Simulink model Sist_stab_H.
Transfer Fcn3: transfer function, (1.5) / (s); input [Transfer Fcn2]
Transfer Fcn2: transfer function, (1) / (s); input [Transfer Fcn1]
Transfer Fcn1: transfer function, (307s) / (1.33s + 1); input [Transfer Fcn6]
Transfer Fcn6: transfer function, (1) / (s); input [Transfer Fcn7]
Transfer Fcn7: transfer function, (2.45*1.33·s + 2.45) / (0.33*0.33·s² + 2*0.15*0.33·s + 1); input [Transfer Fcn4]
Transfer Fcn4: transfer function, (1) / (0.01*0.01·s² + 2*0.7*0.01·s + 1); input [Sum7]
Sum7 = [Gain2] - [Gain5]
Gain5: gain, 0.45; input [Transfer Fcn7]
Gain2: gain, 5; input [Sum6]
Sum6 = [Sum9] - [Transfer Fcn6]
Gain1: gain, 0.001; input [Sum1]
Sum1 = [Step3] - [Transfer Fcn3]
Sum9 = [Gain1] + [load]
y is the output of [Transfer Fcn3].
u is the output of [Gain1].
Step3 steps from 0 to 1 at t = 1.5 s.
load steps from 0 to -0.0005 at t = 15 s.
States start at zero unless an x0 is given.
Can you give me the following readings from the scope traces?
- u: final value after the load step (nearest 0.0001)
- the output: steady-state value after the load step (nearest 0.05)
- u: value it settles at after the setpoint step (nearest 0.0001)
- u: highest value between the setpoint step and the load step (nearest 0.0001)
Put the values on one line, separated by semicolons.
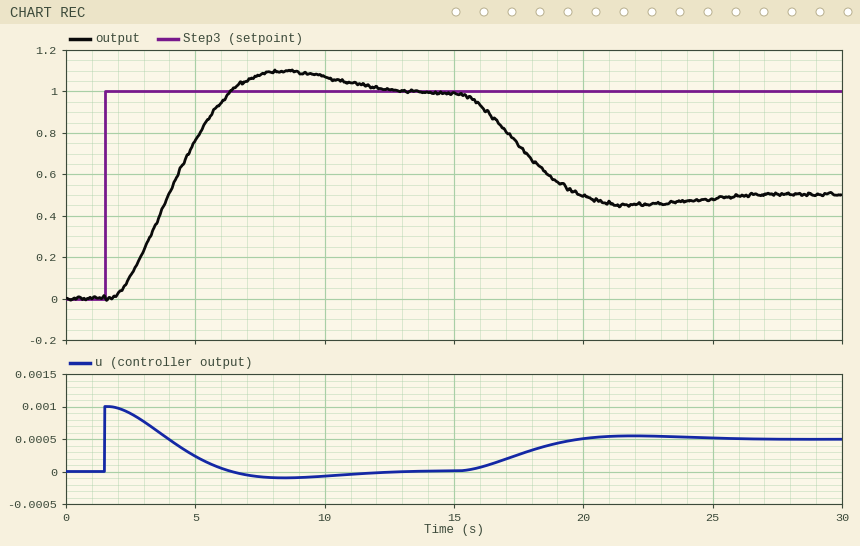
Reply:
0.0005; 0.50; 0.0000; 0.0010
